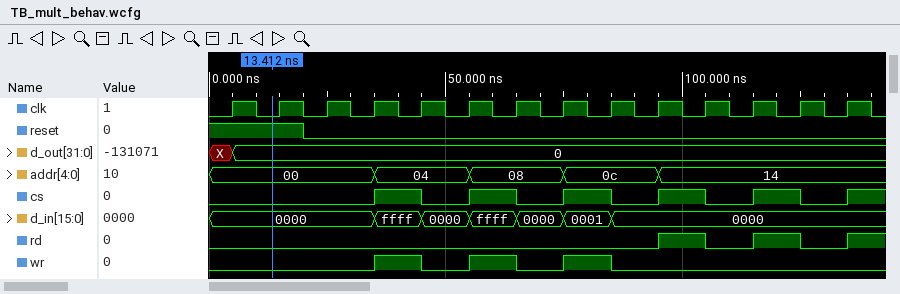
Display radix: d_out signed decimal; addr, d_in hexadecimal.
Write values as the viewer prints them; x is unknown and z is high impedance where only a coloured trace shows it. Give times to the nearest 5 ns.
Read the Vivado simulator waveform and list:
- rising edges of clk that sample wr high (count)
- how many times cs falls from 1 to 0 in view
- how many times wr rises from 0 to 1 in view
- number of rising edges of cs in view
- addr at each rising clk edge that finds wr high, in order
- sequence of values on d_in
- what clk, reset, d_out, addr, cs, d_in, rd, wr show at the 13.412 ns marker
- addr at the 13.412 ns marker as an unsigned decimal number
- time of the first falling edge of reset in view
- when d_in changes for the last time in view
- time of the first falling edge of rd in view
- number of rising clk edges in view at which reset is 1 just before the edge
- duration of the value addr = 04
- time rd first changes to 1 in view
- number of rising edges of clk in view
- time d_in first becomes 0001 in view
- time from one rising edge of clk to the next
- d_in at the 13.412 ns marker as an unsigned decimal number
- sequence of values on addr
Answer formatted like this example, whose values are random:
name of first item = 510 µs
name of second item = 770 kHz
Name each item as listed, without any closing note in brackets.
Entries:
rising edges of clk that sample wr high = 3
how many times cs falls from 1 to 0 in view = 5
how many times wr rises from 0 to 1 in view = 3
number of rising edges of cs in view = 6
addr at each rising clk edge that finds wr high, in order = 04, 08, 0c
sequence of values on d_in = 0000, ffff, 0000, ffff, 0000, 0001, 0000
what clk, reset, d_out, addr, cs, d_in, rd, wr show at the 13.412 ns marker = clk=0, reset=1, d_out=0, addr=00, cs=0, d_in=0000, rd=0, wr=0
addr at the 13.412 ns marker as an unsigned decimal number = 0
time of the first falling edge of reset in view = 20 ns
when d_in changes for the last time in view = 85 ns
time of the first falling edge of rd in view = 105 ns
number of rising clk edges in view at which reset is 1 just before the edge = 2
duration of the value addr = 04 = 20 ns
time rd first changes to 1 in view = 95 ns
number of rising edges of clk in view = 14
time d_in first becomes 0001 in view = 75 ns
time from one rising edge of clk to the next = 10 ns
d_in at the 13.412 ns marker as an unsigned decimal number = 0
sequence of values on addr = 00, 04, 08, 0c, 14
